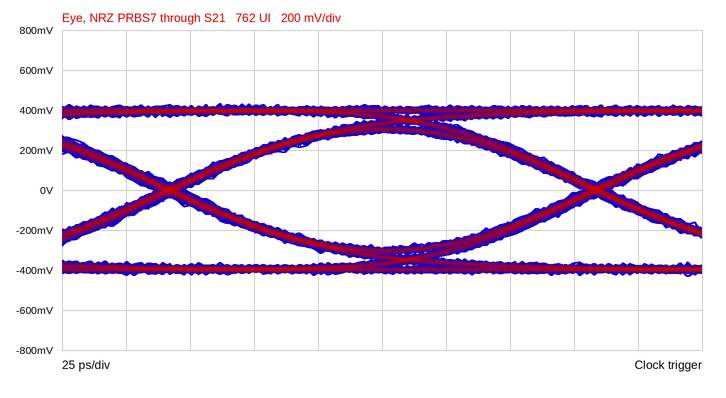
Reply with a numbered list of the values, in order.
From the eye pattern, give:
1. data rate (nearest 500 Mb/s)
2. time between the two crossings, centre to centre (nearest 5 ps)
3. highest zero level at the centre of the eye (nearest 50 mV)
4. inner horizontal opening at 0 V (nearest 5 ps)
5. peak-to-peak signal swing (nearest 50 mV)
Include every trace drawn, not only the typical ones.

1. 6.0 Gb/s
2. 165 ps
3. -300 mV
4. 155 ps
5. 850 mV
